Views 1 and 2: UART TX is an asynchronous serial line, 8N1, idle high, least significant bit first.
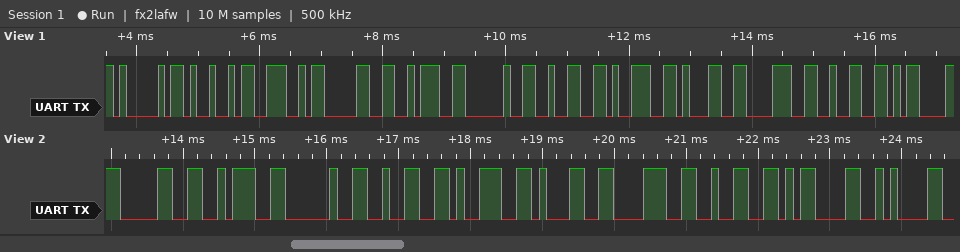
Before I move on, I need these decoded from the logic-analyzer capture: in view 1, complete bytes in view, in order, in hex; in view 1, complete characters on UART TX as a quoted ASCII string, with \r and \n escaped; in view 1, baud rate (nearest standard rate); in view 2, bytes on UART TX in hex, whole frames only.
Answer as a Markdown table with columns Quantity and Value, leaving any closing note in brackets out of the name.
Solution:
| Quantity | Value |
|---|---|
| in view 1, complete bytes in view, in order, in hex | 41 49 4E 30 3A 20 32 39 31 38 32 0D |
| in view 1, complete characters on UART TX as a quoted ASCII string, with \r and \n escaped | "AIN0: 29182\r" |
| in view 1, baud rate | 9600 baud |
| in view 2, bytes on UART TX in hex, whole frames only | 30 3A 20 32 39 31 38 32 0D 0A |
